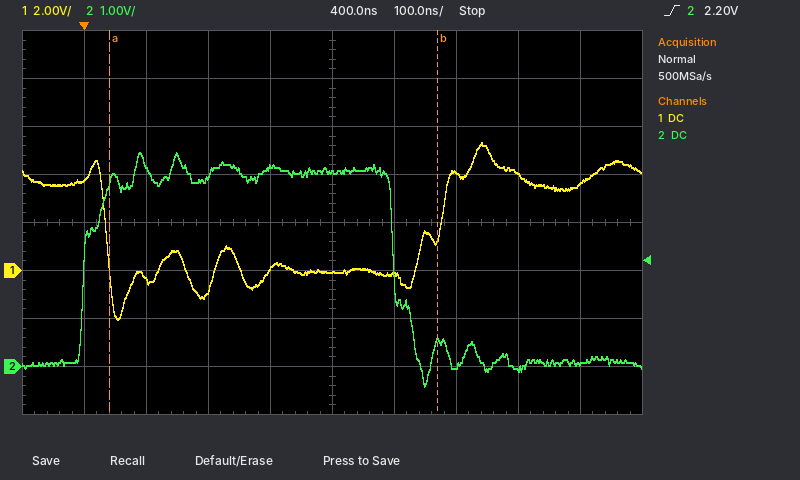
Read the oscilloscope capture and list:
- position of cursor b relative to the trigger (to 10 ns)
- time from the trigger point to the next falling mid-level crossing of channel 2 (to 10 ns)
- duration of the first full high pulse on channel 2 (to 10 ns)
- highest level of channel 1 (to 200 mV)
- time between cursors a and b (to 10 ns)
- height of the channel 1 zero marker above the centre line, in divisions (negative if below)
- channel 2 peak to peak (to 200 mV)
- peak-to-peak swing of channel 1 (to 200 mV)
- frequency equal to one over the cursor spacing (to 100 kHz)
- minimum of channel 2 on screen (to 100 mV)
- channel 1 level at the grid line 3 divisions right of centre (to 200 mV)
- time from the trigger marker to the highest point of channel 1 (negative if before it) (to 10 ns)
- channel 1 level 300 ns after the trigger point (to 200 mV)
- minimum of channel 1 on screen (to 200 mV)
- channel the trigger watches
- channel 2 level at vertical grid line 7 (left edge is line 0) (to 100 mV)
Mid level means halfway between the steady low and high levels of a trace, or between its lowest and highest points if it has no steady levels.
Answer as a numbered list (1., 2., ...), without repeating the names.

1. +570 ns
2. 500 ns
3. 500 ns
4. 5.4 V
5. 530 ns
6. -1.0 div
7. 4.8 V
8. 7.4 V
9. 1.9 MHz
10. -400 mV
11. 4.0 V
12. +640 ns
13. 0.0 V
14. -2.0 V
15. channel 2
16. 0.0 V
